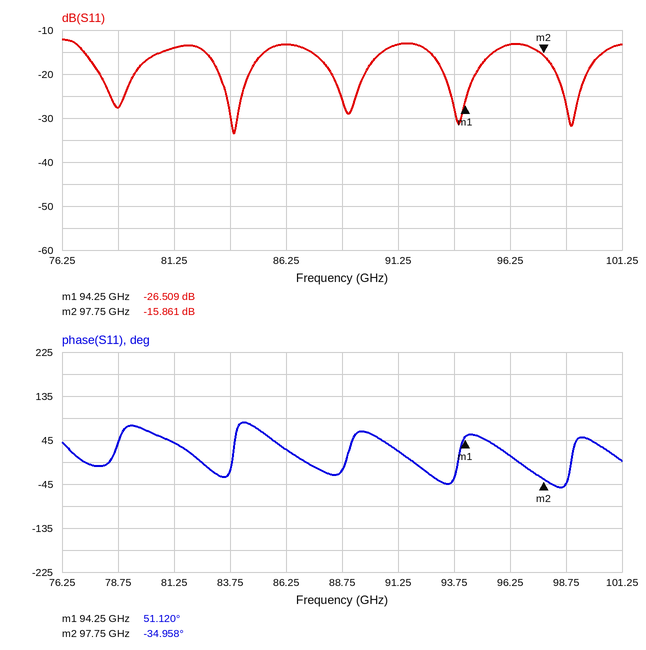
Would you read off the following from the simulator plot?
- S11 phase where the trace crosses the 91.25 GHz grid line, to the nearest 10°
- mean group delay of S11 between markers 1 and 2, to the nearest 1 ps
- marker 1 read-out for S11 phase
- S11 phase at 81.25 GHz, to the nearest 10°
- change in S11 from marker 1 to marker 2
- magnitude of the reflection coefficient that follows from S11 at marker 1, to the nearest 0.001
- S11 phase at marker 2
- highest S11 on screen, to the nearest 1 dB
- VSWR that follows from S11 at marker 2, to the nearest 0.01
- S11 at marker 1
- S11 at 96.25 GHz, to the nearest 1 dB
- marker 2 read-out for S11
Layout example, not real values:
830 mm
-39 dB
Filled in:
20°
68 ps
51.120°
40°
10.648 dB
0.047
-34.958°
-12 dB
1.38
-26.509 dB
-13 dB
-15.861 dB
